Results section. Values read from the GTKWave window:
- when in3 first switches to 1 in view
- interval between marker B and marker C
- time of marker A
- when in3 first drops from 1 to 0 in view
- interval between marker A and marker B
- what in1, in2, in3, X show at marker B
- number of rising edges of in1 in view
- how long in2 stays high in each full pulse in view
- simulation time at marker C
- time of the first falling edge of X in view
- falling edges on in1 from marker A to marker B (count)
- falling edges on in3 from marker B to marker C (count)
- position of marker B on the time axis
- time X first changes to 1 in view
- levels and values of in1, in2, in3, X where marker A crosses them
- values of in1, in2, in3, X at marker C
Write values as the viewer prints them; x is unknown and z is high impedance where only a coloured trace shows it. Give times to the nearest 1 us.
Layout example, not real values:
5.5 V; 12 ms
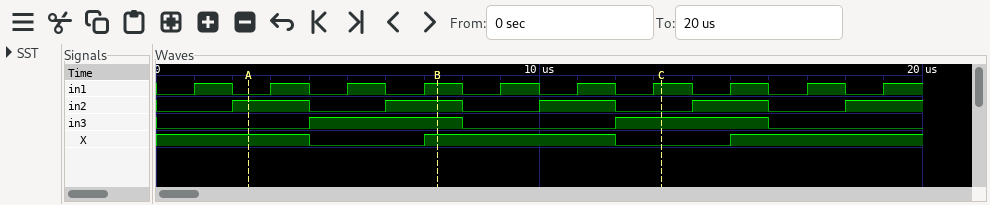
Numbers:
4 us; 6 us; 2 us; 8 us; 5 us; in1=1, in2=1, in3=1, X=1; 10; 2 us, 2 us, 2 us, 2 us; 13 us; 4 us; 2; 1; 7 us; 7 us; in1=0, in2=1, in3=0, X=1; in1=1, in2=0, in3=1, X=0
